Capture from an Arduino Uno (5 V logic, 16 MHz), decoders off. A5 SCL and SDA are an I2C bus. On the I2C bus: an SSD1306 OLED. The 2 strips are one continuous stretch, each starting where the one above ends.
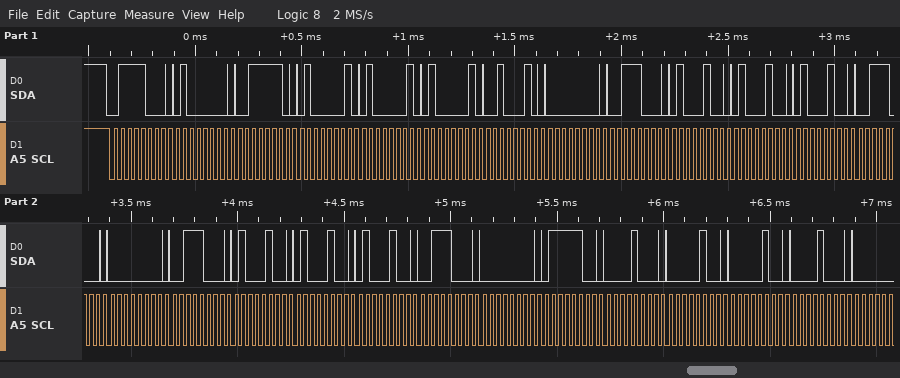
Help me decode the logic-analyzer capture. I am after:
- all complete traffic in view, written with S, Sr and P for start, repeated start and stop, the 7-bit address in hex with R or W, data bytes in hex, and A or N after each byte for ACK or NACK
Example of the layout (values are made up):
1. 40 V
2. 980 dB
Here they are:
1. S 3CW A 40 A 3E A 41 A 41 A 41 A 22 A 00 A 38 A 44 A 44 A 44 A 38 A 00 A 38 A 44 A 44 A 44 A 38 A 00 A 7C A 08 A 04 A 04 A 08 A
